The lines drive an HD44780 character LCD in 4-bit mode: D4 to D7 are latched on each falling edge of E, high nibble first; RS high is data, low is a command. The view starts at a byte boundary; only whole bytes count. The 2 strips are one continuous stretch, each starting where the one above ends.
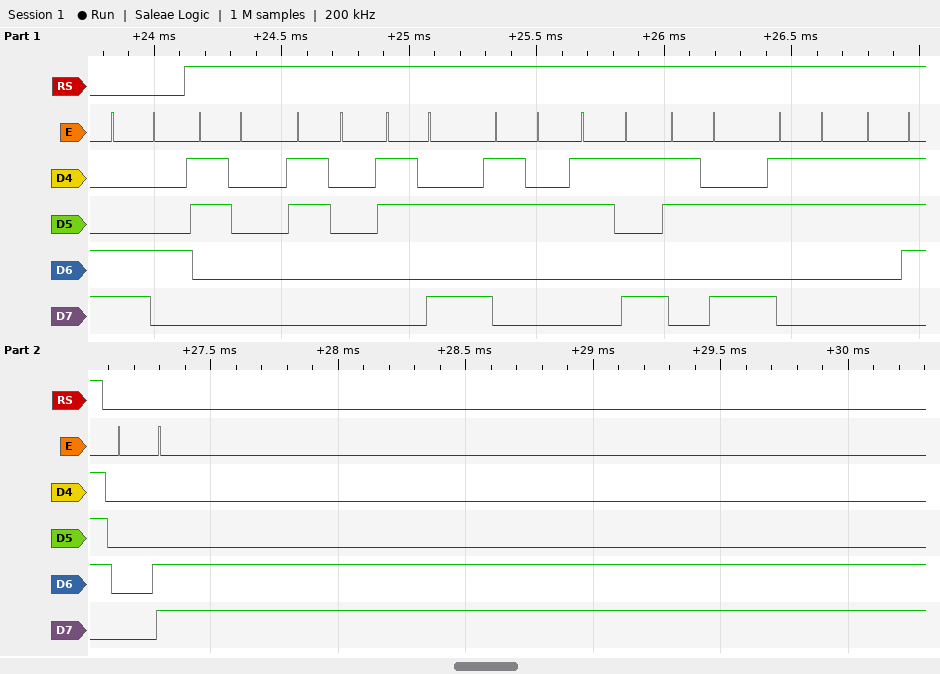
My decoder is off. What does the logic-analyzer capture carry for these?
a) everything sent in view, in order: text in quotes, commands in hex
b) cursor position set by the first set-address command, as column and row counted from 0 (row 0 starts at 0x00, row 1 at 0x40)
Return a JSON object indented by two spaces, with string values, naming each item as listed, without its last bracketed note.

{
  "everything sent in view, in order: text in quotes, commands in hex": "0xC4 \"00:29:37\" 0x0C",
  "cursor position set by the first set-address command, as column and row counted from 0": "column 4, row 1"
}
